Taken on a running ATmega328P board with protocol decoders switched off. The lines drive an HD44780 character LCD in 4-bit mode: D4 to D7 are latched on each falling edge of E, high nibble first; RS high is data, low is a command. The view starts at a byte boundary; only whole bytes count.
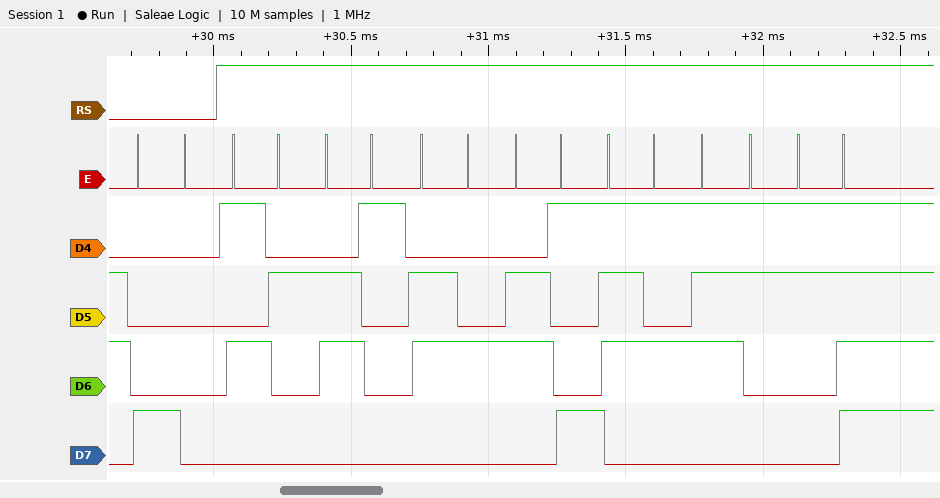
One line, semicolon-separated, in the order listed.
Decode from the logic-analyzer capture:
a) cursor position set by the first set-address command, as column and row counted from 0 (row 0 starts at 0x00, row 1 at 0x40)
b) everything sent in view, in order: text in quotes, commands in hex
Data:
column 0, row 0; 0x80 "Radius?"
